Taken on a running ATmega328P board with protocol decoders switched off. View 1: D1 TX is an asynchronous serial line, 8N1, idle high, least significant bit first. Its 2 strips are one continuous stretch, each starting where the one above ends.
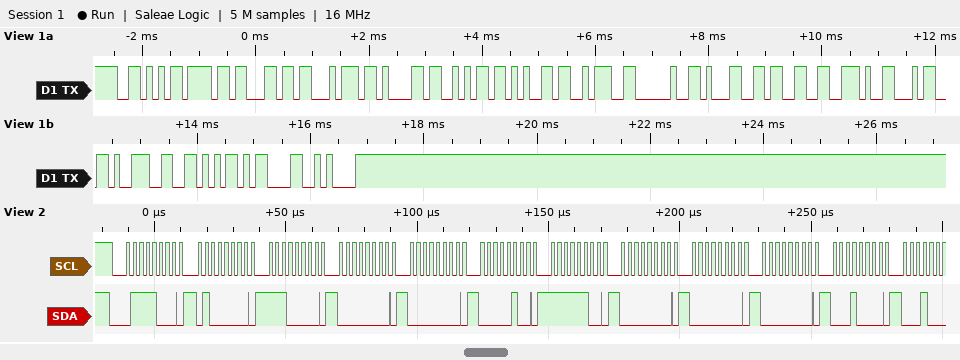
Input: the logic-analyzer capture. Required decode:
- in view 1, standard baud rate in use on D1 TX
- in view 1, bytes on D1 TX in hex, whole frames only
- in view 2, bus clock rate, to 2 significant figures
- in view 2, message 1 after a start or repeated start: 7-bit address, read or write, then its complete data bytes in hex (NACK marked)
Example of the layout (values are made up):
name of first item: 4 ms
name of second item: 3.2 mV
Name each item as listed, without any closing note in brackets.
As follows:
in view 1, standard baud rate in use on D1 TX: 9600 baud
in view 1, bytes on D1 TX in hex, whole frames only: 56 6F 6C 74 61 6A 65 3A 20 31 33 2E 34 39 56 0D 0A
in view 2, bus clock rate, to 2 significant figures: 400 kHz
in view 2, message 1 after a start or repeated start: 7-bit address, read or write, then its complete data bytes in hex: 0x3C write: 40 E0 00 00 04 FC 00 00 00 10
